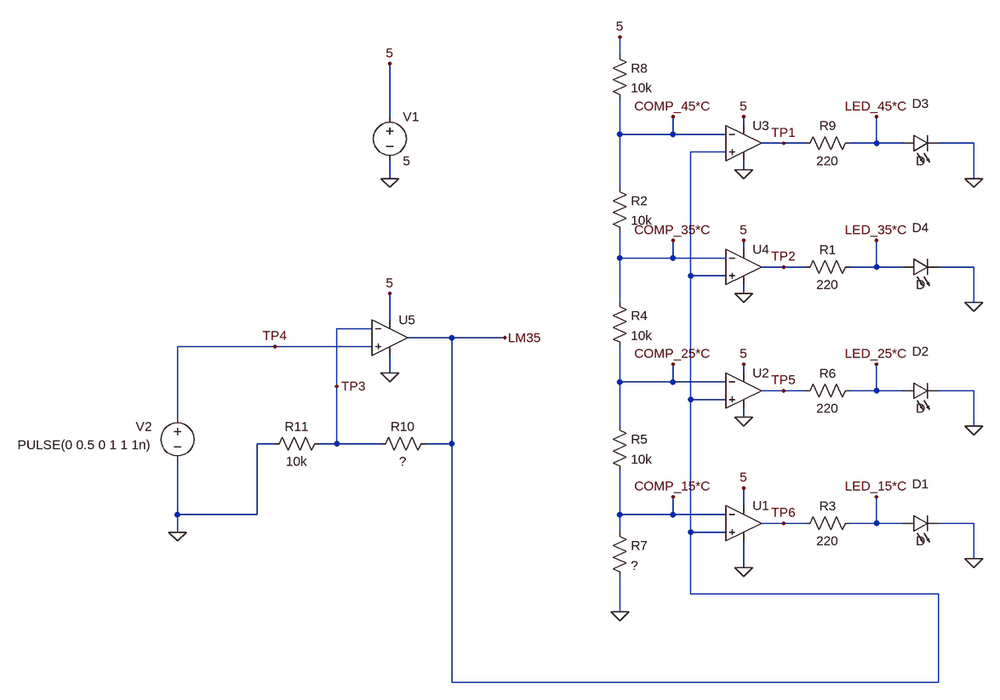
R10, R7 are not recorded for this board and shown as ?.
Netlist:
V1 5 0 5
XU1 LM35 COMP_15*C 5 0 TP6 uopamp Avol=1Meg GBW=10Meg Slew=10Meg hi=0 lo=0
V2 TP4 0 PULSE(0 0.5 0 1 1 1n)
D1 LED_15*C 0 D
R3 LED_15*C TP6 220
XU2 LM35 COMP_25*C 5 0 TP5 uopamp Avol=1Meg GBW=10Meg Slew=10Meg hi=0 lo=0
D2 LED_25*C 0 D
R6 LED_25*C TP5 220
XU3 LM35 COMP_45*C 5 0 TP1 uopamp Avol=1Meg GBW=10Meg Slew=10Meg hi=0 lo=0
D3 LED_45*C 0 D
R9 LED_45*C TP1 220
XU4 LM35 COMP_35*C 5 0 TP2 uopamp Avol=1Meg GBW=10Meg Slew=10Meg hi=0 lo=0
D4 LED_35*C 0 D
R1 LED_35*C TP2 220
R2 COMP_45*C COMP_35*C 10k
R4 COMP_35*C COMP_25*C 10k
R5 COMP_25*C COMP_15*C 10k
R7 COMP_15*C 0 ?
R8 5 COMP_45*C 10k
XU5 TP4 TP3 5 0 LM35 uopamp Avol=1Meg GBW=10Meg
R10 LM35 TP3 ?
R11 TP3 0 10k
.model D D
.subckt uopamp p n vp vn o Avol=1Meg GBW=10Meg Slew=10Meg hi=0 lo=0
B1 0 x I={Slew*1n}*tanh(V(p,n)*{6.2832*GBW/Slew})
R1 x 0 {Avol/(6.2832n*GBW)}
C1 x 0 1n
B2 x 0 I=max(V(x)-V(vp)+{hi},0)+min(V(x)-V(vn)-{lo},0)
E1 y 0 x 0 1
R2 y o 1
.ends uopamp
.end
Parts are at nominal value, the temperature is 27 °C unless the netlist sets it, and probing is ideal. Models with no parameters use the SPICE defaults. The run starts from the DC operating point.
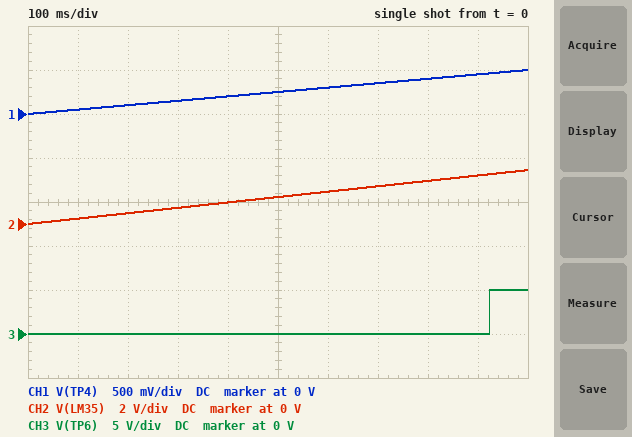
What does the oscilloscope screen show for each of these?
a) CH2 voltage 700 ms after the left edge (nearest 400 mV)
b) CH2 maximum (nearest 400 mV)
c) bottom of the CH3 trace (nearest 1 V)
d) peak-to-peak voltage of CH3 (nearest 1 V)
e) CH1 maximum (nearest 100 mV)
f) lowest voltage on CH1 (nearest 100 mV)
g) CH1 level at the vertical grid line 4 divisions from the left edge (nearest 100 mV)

1.6 V
2.4 V
0 V
5 V
500 mV
0 V
200 mV
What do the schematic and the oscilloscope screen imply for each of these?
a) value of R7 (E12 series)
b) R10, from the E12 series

33 kΩ
39 kΩ
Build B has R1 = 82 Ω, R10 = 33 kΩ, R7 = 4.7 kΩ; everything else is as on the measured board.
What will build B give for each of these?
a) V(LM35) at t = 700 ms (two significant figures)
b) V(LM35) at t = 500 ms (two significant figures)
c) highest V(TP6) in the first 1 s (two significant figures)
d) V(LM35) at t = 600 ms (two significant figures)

1.5 V
1.1 V
5.0 V
1.3 V
